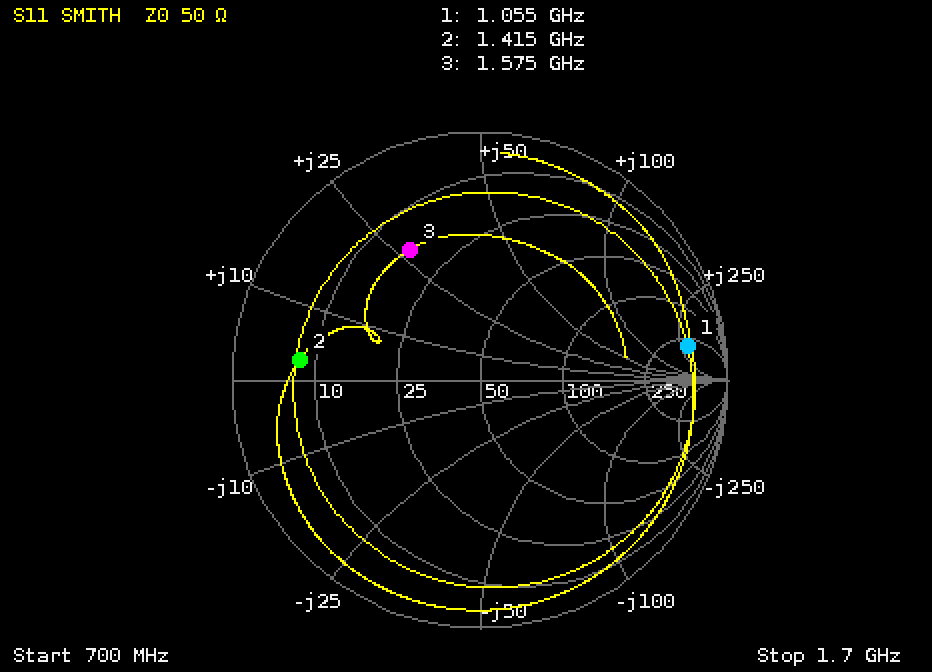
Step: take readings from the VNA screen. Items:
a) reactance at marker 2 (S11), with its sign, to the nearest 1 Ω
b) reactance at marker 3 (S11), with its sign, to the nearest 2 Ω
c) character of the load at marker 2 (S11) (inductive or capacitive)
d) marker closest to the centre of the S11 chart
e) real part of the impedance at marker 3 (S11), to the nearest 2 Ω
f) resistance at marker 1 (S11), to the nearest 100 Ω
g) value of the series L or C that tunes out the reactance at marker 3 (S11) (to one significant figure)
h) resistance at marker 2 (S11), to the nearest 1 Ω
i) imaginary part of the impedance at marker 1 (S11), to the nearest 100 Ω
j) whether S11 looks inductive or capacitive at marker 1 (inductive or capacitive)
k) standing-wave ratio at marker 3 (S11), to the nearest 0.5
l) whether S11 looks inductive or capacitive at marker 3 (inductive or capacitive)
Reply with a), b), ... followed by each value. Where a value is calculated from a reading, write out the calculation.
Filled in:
a) +3 Ω
b) +28 Ω
c) inductive
d) marker 3
e) 16 Ω
f) 300 Ω
g) C = 1/(2π × 1.575 GHz × 28 Ω) ≈ 4 pF
h) 8 Ω
i) +300 Ω
j) inductive
k) 4.0
l) inductive
